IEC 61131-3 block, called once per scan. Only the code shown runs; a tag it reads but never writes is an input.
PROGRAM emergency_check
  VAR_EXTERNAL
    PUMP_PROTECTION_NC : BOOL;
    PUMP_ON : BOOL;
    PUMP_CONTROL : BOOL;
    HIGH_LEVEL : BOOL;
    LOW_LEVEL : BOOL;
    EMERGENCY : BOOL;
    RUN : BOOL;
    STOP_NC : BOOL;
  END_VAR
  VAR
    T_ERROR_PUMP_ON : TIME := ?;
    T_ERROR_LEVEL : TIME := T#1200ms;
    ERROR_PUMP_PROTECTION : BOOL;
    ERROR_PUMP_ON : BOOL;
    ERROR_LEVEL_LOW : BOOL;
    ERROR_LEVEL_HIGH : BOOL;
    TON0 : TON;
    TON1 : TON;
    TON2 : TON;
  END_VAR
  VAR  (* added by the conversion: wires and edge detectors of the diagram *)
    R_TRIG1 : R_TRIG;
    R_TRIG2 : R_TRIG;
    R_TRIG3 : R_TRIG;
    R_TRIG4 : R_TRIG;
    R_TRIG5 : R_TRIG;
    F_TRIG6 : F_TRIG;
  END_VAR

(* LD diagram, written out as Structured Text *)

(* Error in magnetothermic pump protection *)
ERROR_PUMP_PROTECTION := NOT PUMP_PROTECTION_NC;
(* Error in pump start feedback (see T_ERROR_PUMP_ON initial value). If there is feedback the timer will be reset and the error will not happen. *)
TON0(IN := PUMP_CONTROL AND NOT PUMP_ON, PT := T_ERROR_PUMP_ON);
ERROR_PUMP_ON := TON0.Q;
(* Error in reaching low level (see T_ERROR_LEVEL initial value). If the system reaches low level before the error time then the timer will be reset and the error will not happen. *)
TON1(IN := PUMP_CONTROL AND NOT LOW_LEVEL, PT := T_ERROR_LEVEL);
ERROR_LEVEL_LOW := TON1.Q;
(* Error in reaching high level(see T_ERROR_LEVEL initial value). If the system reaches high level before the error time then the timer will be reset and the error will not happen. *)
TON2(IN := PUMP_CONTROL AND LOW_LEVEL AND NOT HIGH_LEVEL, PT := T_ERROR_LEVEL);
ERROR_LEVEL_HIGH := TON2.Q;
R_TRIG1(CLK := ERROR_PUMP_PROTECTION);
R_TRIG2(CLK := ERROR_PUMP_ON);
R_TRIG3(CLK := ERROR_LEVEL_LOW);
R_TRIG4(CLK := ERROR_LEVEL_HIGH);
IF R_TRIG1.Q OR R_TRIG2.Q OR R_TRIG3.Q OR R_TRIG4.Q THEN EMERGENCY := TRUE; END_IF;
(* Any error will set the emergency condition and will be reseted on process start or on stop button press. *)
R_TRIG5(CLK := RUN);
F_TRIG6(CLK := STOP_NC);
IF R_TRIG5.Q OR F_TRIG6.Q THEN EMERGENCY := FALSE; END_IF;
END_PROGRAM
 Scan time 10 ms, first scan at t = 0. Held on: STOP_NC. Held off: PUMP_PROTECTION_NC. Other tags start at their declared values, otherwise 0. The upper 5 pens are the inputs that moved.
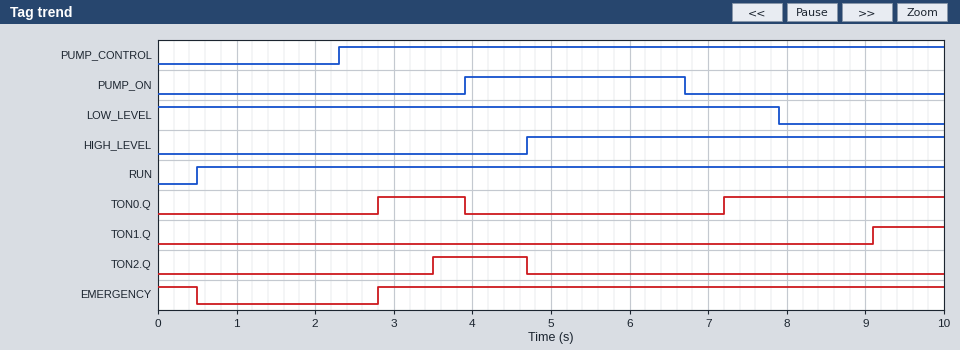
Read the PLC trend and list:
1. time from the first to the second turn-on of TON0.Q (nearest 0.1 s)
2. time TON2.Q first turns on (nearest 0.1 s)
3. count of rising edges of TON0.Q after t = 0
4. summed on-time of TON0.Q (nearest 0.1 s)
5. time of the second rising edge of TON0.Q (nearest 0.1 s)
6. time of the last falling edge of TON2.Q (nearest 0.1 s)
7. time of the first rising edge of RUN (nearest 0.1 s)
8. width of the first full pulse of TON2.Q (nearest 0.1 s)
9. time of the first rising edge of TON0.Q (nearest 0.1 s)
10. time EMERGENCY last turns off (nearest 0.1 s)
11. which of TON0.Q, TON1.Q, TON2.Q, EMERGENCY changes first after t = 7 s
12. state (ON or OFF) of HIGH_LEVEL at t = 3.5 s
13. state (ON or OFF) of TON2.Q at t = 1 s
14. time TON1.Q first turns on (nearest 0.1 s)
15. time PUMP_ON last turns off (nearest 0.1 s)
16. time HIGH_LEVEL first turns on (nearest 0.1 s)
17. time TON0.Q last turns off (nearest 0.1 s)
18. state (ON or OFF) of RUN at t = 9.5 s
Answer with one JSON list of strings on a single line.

["4.4 s", "3.5 s", "2", "3.9 s", "7.2 s", "4.7 s", "0.5 s", "1.2 s", "2.8 s", "0.5 s", "TON0.Q", "OFF", "OFF", "9.1 s", "6.7 s", "4.7 s", "3.9 s", "ON"]
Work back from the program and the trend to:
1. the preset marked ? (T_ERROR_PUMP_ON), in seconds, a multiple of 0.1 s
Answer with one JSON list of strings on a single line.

["0.5 s"]
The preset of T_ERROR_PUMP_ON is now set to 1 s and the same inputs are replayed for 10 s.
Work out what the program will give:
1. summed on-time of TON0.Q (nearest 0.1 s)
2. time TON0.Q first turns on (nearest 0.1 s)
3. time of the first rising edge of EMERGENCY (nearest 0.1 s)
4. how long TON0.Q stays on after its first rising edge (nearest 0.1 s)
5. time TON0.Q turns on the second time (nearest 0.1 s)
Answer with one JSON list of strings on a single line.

["2.9 s", "3.3 s", "3.3 s", "0.6 s", "7.7 s"]
